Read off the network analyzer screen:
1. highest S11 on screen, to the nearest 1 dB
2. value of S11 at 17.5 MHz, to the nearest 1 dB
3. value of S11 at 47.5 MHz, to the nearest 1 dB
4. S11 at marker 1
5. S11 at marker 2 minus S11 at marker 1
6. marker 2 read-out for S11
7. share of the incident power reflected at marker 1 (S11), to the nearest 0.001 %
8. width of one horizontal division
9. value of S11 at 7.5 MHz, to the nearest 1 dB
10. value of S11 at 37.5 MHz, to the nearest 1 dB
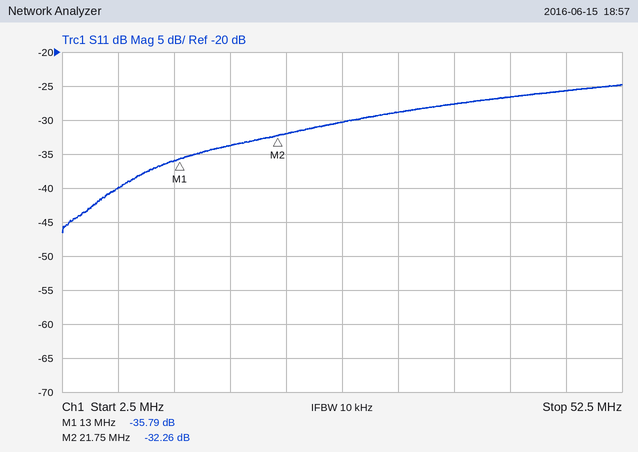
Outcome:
-25 dB
-34 dB
-26 dB
-35.79 dB
3.53 dB
-32.26 dB
0.026 %
5 MHz
-40 dB
-28 dB
